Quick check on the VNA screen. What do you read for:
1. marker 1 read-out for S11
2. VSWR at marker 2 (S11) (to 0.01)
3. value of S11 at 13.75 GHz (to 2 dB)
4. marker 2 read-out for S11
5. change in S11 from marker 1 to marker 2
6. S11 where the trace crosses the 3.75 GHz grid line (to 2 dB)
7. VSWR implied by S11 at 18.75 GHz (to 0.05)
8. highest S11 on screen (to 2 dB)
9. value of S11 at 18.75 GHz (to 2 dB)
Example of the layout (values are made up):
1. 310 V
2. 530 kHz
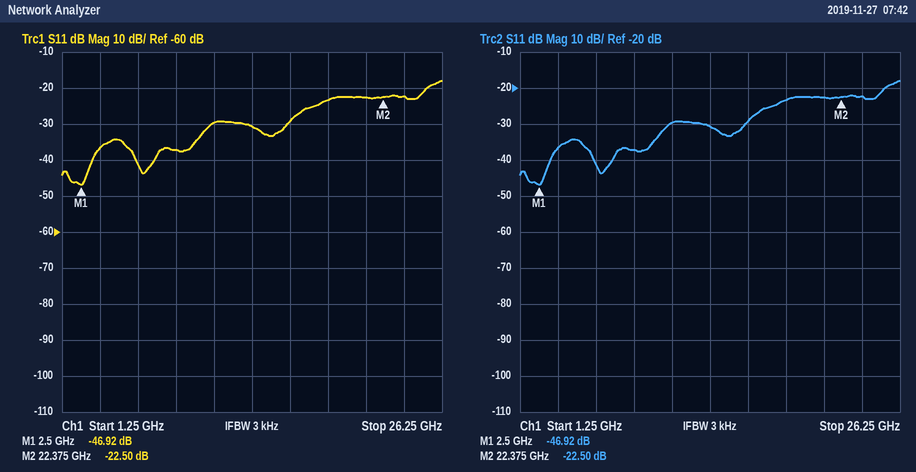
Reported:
1. -46.92 dB
2. 1.16
3. -30 dB
4. -22.50 dB
5. 24.42 dB
6. -36 dB
7. 1.15
8. -18 dB
9. -24 dB
